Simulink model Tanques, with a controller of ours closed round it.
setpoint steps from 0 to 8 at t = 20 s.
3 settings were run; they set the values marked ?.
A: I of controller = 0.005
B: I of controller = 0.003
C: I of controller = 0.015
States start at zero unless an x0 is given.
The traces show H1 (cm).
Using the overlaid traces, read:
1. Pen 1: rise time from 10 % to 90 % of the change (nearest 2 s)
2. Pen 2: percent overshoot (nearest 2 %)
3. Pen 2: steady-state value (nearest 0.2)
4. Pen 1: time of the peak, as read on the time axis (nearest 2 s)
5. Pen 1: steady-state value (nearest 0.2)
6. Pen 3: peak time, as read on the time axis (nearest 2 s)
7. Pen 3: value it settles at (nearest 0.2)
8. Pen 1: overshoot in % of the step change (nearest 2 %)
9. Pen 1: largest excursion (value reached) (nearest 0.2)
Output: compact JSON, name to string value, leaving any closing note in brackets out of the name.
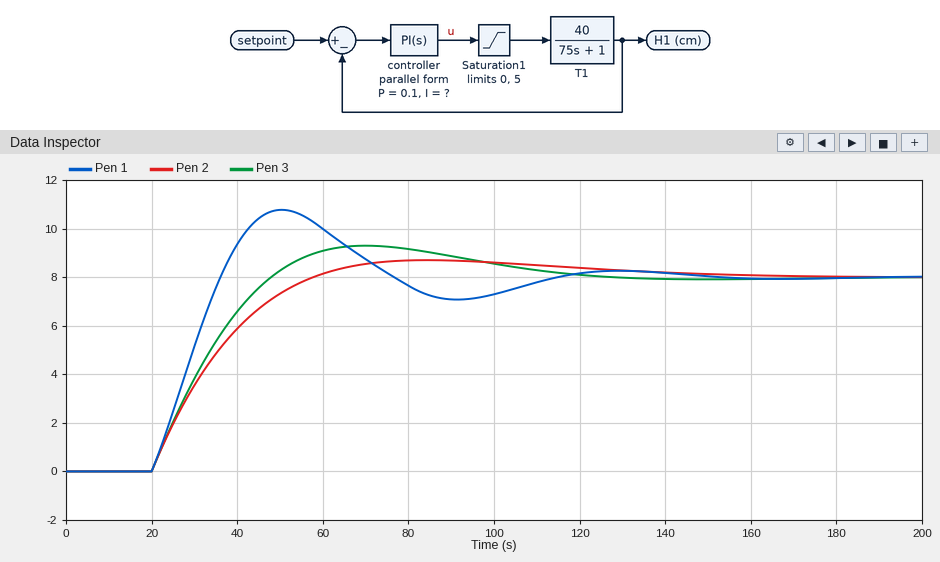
{"Pen 1: rise time from 10 % to 90 % of the change": "12 s", "Pen 2: percent overshoot": "8 %", "Pen 2: steady-state value": "8.0", "Pen 1: time of the peak, as read on the time axis": "50 s", "Pen 1: steady-state value": "8.0", "Pen 3: peak time, as read on the time axis": "70 s", "Pen 3: value it settles at": "8.0", "Pen 1: overshoot in % of the step change": "34 %", "Pen 1: largest excursion (value reached)": "10.8"}
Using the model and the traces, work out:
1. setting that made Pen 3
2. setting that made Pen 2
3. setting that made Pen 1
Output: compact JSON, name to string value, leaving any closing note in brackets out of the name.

{"setting that made Pen 3": "A", "setting that made Pen 2": "B", "setting that made Pen 1": "C"}
